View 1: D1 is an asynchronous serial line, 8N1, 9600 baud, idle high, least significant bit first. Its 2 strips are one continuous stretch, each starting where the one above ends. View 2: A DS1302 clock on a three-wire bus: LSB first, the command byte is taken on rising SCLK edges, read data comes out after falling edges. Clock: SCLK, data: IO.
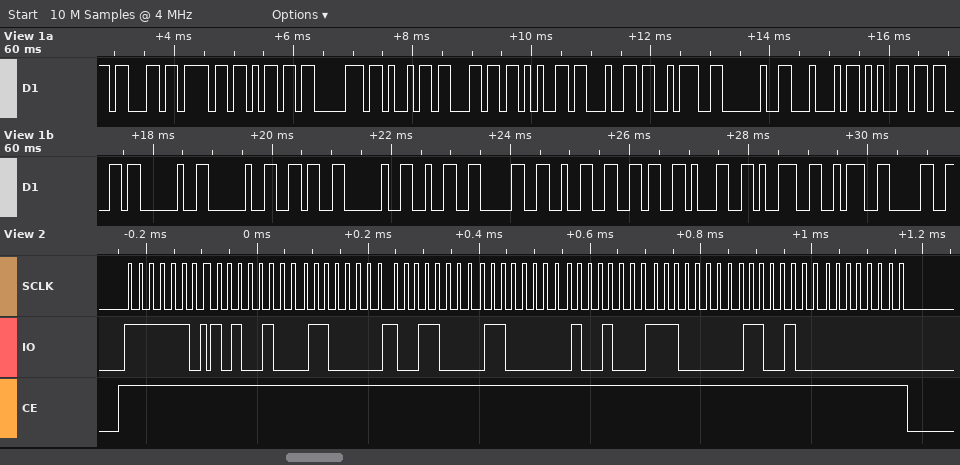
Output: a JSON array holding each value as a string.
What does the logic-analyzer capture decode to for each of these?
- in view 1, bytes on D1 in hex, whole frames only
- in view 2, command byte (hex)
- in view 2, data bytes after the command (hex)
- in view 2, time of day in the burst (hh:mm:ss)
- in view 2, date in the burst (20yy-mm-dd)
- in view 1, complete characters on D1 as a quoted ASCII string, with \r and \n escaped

["63 6F 6D 70 69 6C 65 64 3A 20 44 65 63 20 20 36 20 32 30 32 36 31 39 3A 30", "0xBF", "25 06 19 06 12 07 26 00", "19:06:25", "2026-12-06", "\"compiled: Dec  6 202619:0\""]
